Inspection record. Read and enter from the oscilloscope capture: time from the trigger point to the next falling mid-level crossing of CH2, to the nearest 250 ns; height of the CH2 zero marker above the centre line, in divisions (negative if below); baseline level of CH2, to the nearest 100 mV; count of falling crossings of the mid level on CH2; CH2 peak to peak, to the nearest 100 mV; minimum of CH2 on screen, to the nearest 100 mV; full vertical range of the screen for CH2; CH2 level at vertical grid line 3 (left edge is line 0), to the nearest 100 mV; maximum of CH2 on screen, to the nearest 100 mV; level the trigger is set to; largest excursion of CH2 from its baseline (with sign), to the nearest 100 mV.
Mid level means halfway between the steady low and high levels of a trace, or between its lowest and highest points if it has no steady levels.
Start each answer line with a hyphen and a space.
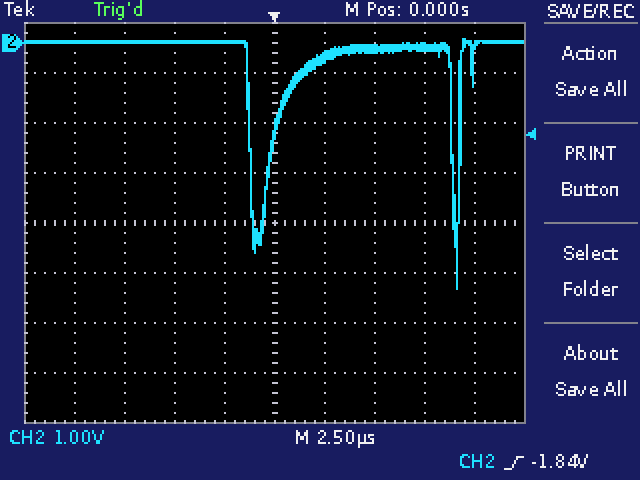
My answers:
- 9.00 µs
- +3.6 div
- 0.0 V
- 2
- 5.0 V
- -4.9 V
- 8 V
- 0.0 V
- 100 mV
- -1.84 V
- -4.9 V
